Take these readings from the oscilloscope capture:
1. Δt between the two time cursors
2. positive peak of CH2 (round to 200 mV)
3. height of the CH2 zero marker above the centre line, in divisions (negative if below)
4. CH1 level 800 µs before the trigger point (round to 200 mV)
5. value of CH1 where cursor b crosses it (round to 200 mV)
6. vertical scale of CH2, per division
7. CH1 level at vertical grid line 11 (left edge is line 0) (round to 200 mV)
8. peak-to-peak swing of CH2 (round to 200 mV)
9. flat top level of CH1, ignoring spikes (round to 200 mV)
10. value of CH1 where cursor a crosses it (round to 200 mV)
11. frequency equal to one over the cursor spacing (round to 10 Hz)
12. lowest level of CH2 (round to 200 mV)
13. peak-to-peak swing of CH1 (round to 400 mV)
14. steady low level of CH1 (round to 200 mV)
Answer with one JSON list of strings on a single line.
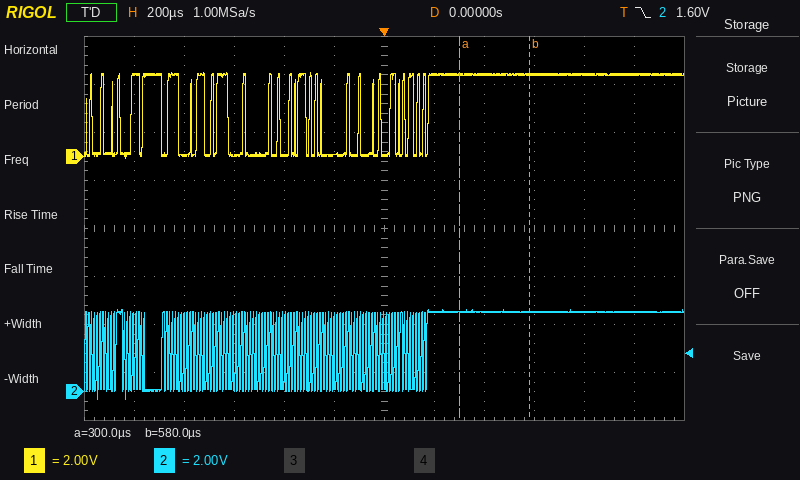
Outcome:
["280 µs", "3.4 V", "-3.4 div", "0.0 V", "3.4 V", "2 V", "3.4 V", "3.8 V", "3.4 V", "3.4 V", "3.57 kHz", "-400 mV", "3.6 V", "0.0 V"]
